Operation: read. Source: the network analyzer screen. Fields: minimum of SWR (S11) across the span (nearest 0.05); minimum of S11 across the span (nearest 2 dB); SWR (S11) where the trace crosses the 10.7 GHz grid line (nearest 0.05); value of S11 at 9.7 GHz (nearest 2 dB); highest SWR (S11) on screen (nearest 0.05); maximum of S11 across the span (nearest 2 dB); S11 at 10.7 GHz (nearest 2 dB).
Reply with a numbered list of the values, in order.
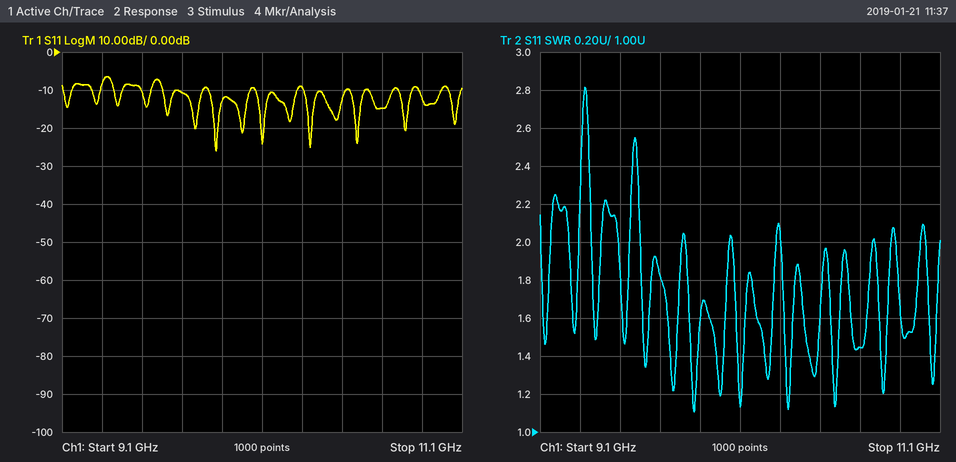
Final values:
1. 1.10
2. -26 dB
3. 1.45
4. -10 dB
5. 2.80
6. -6 dB
7. -14 dB
